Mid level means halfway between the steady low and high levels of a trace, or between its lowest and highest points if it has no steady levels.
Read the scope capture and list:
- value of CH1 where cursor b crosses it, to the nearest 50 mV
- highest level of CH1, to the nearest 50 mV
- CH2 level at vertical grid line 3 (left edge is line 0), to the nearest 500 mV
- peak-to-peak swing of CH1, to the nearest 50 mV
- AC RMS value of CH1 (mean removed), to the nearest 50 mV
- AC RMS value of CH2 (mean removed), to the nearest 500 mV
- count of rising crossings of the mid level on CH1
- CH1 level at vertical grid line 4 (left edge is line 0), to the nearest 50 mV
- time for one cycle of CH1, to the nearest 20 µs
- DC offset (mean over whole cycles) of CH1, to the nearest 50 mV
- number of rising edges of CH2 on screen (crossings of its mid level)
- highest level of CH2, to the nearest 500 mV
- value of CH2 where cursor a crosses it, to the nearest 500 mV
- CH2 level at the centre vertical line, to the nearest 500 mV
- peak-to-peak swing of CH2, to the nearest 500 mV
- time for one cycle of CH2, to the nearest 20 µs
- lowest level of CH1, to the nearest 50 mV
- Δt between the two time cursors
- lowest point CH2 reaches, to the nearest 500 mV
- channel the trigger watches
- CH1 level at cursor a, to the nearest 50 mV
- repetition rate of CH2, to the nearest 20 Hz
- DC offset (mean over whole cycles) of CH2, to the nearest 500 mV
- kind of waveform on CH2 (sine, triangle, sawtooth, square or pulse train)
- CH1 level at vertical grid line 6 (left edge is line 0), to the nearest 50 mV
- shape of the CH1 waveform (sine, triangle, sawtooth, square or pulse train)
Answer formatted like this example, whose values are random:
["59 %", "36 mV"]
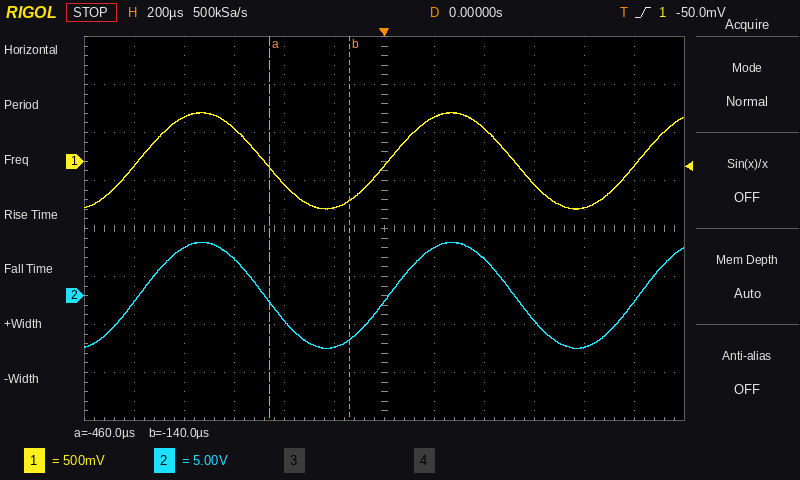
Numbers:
["-400 mV", "500 mV", "4.0 V", "1.00 V", "350 mV", "4.0 V", "3", "-250 mV", "1.00 ms", "0 mV", "3", "5.5 V", "-500 mV", "-500 mV", "11.0 V", "1.00 ms", "-500 mV", "320 µs", "-5.5 V", "CH1", "-50 mV", "1.00 kHz", "0.0 V", "sine", "-50 mV", "sine"]
